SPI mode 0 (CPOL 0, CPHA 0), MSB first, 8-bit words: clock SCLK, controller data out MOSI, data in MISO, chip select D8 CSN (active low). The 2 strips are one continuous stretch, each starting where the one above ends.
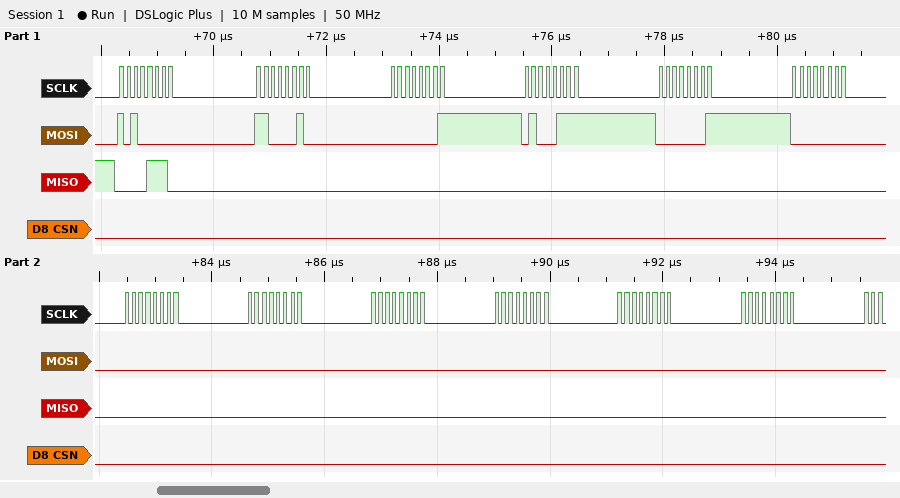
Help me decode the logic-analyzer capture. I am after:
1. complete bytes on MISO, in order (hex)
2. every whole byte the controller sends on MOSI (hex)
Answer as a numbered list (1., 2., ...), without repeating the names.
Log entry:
1. 0E 00 00 00 00 00 00 00 00 00 00 00
2. A0 C2 01 47 01 00 00 00 00 00 00 00
